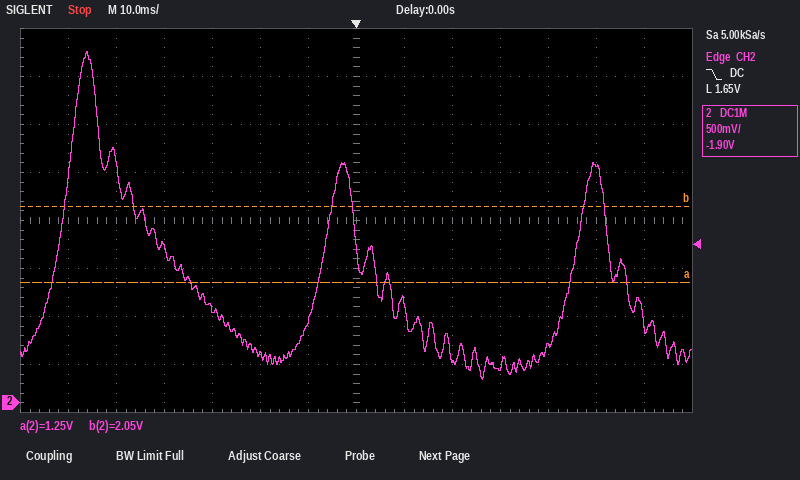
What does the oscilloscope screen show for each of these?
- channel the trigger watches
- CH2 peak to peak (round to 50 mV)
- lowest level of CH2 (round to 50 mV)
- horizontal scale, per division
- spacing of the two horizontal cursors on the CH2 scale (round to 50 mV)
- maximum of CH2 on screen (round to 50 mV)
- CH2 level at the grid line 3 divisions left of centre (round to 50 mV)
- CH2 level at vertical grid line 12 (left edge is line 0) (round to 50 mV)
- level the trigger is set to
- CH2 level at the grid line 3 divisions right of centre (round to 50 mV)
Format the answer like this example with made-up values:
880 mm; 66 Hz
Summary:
CH2; 3.40 V; 250 mV; 10 ms; 800 mV; 3.65 V; 1.00 V; 2.45 V; 1.65 V; 400 mV
